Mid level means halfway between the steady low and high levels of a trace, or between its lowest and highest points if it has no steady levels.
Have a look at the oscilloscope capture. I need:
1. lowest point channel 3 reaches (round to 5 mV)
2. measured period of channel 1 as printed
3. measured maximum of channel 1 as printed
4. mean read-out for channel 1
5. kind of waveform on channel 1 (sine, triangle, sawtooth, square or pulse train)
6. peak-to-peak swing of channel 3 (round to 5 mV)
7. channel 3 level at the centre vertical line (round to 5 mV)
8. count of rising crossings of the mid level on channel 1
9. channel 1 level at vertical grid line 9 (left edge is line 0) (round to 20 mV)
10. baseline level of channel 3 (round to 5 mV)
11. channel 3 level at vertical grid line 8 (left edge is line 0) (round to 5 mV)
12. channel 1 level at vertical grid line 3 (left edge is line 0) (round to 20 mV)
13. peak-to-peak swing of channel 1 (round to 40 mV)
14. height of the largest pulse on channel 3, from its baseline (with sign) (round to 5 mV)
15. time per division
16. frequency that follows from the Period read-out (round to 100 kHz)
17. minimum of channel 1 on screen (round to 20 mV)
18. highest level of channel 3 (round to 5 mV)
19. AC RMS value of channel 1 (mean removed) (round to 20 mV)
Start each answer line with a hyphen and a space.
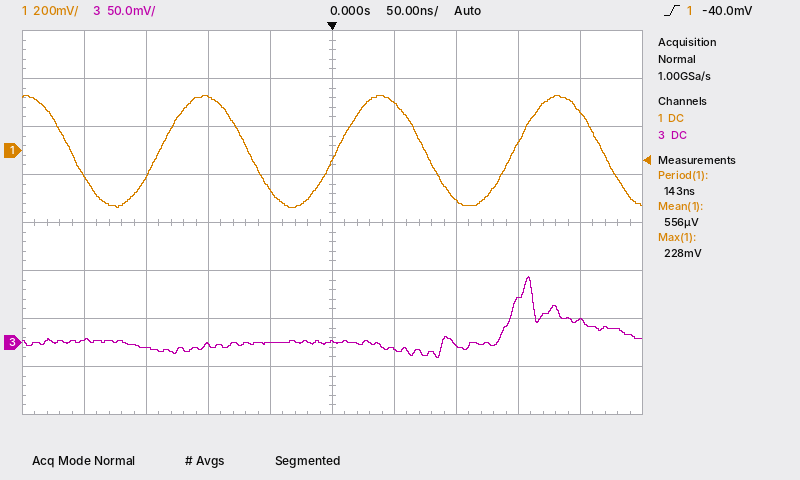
- -15 mV
- 143 ns
- 228 mV
- 556 µV
- sine
- 85 mV
- 0 mV
- 3
- 160 mV
- 0 mV
- 45 mV
- 220 mV
- 480 mV
- +70 mV
- 50 ns
- 7.0 MHz
- -240 mV
- 70 mV
- 160 mV
